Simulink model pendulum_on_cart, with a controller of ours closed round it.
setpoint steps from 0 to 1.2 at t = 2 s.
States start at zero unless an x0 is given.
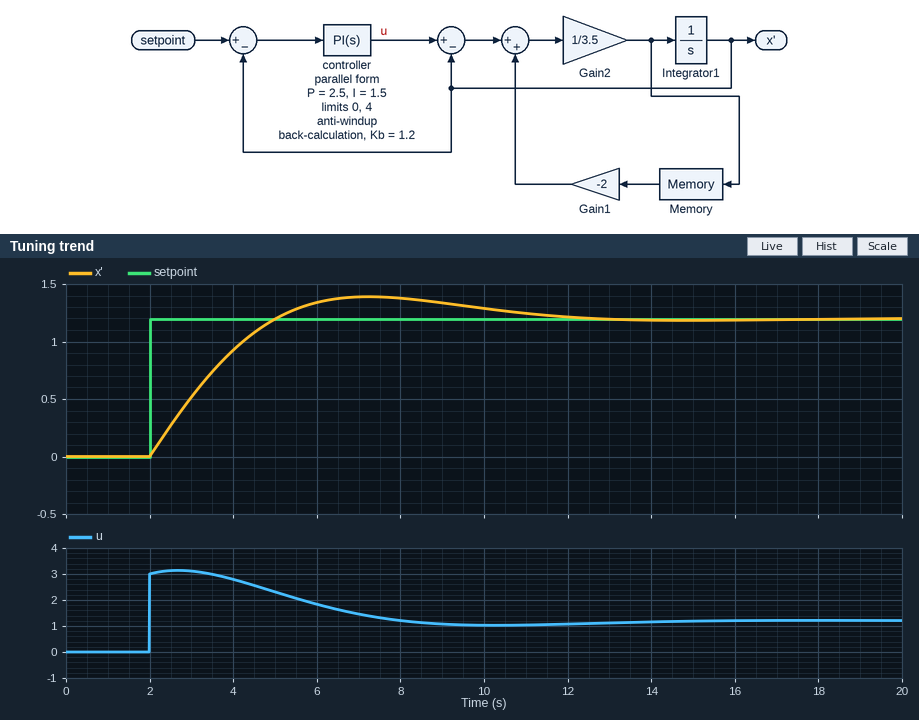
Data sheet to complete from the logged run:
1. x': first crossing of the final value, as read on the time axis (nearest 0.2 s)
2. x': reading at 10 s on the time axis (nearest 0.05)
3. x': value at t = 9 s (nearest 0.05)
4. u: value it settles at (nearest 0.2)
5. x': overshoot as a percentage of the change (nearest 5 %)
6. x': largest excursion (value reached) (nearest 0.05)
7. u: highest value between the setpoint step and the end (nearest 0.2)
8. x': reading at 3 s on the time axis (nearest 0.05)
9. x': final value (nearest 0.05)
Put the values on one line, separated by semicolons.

5.0 s; 1.30; 1.35; 1.2; 15 %; 1.40; 3.2; 0.50; 1.20
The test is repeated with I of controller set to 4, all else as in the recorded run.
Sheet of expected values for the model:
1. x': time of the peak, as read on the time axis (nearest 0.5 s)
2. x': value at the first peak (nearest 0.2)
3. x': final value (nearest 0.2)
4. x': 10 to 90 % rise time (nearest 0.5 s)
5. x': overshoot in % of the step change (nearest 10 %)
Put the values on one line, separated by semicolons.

5.5 s; 1.6; 1.2; 1.5 s; 30 %
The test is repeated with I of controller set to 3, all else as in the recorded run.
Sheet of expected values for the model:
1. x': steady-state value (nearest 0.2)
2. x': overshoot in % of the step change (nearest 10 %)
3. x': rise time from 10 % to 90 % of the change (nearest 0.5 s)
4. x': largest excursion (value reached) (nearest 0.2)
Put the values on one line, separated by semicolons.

1.2; 30 %; 1.5 s; 1.6
